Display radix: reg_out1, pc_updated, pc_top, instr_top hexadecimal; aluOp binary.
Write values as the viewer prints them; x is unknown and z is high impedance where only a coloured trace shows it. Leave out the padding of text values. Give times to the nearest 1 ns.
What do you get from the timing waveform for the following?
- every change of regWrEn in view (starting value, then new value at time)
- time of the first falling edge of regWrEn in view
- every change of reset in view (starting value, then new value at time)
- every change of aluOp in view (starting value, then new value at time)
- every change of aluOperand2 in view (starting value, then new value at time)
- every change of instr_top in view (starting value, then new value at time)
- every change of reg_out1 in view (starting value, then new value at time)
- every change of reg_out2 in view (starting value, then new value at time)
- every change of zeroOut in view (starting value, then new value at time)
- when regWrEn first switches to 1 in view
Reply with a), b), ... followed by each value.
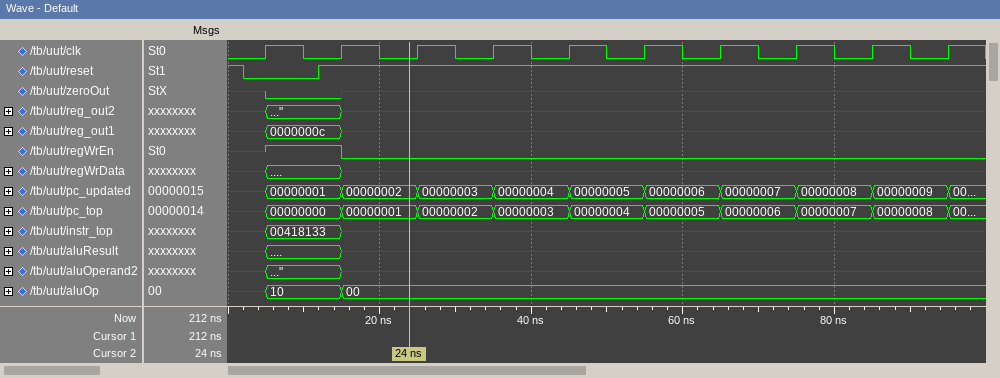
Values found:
a) x, 1 at 5 ns, 0 at 15 ns
b) 15 ns
c) 1, 0 at 2 ns, 1 at 12 ns
d) x, 10 at 5 ns, 00 at 15 ns
e) x, " at 5 ns, x at 15 ns
f) x, 00418133 at 5 ns, x at 15 ns
g) x, 0000000c at 5 ns, x at 15 ns
h) x, " at 5 ns, x at 15 ns
i) x, 0 at 5 ns, x at 15 ns
j) 5 ns
